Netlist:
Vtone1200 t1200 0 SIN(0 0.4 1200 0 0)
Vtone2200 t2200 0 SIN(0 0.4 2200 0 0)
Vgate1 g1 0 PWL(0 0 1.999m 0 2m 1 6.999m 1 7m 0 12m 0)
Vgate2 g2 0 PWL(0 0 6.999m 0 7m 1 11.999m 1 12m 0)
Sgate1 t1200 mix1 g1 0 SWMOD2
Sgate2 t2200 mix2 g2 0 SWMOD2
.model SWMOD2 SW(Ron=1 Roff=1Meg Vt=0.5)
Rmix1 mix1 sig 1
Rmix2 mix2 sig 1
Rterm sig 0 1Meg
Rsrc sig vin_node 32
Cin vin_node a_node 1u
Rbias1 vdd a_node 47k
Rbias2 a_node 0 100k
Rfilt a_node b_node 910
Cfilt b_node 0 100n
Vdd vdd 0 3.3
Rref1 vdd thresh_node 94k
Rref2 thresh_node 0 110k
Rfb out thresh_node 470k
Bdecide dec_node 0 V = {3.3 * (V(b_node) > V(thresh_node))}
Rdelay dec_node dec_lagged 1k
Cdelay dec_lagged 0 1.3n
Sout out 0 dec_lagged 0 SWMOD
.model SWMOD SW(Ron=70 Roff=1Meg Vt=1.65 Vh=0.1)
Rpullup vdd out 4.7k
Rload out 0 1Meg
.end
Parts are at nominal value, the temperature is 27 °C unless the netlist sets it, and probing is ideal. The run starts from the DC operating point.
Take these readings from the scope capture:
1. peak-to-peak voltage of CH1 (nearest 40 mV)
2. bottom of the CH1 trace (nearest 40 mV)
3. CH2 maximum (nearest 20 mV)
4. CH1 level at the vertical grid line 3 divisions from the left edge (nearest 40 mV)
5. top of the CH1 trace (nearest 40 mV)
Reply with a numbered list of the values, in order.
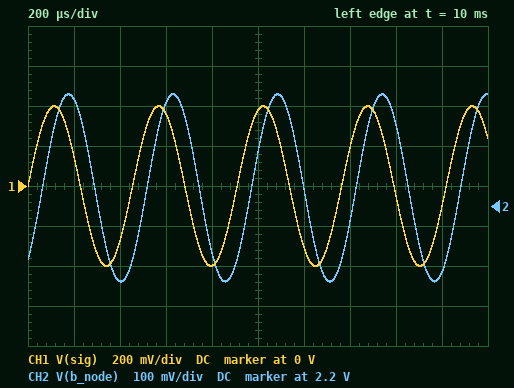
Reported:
1. 800 mV
2. -400 mV
3. 2.48 V
4. 360 mV
5. 400 mV
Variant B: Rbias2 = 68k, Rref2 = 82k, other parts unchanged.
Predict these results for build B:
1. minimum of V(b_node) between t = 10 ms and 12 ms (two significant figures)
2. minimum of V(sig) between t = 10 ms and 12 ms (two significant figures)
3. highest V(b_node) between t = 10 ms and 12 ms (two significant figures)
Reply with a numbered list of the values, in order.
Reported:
1. 1.7 V
2. -400 mV
3. 2.2 V
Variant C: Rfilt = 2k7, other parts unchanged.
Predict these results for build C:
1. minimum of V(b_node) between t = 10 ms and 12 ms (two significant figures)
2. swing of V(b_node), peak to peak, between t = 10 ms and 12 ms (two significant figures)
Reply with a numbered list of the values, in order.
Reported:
1. 2.1 V
2. 200 mV
